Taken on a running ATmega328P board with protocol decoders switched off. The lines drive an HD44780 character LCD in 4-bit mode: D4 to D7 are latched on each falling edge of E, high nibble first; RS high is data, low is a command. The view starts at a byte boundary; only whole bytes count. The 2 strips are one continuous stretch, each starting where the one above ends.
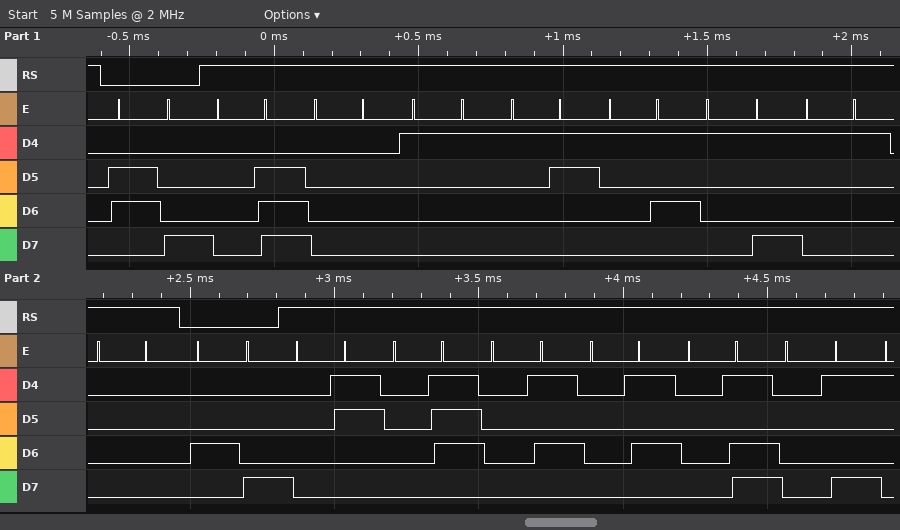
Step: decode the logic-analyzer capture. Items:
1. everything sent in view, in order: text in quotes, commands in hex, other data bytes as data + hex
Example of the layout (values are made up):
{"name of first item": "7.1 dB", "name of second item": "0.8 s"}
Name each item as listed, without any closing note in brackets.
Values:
{"everything sent in view, in order: text in quotes, commands in hex, other data bytes as data + hex": "0x68 data 0E 00 11 13 15 19 11 00 0x48 data 03 07 05 05 0D 09"}
